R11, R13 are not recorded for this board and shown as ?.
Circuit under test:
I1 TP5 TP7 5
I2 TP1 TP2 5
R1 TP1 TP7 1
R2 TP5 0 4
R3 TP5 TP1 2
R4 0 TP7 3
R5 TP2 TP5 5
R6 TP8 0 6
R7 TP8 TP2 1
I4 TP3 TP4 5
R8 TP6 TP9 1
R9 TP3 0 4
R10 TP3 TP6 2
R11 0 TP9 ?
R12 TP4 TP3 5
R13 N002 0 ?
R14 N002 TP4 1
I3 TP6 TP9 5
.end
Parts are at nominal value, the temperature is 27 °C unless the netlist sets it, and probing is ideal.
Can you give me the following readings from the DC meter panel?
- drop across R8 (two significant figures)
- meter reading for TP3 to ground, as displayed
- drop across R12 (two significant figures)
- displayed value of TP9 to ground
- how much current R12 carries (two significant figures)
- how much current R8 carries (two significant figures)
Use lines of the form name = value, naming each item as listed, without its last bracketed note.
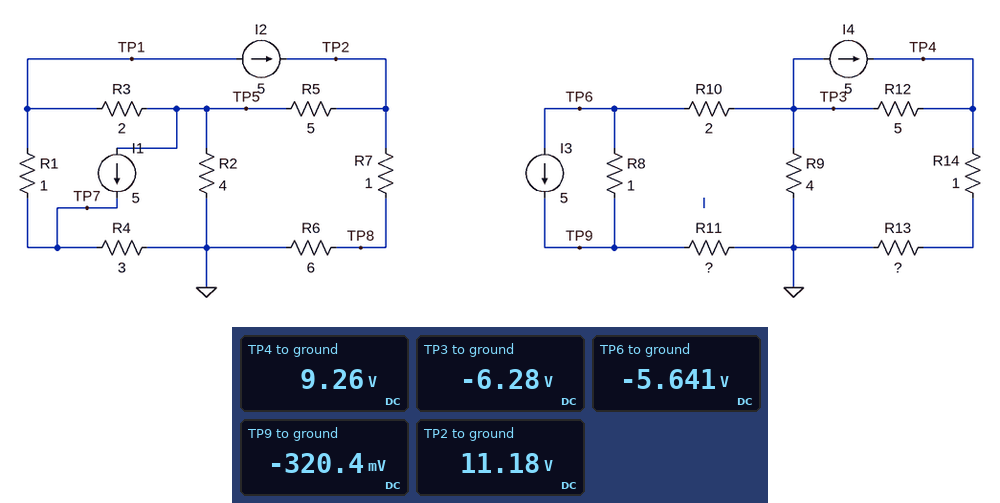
drop across R8 = 5.3 V
meter reading for TP3 to ground, as displayed = -6.28 V
drop across R12 = 16 V
displayed value of TP9 to ground = -320.4 mV
how much current R12 carries = 3.1 A
how much current R8 carries = 5.3 A
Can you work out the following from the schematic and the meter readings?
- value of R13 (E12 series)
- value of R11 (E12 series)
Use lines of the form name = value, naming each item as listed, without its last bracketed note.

value of R13 = 3.9 Ω
value of R11 = 1 Ω
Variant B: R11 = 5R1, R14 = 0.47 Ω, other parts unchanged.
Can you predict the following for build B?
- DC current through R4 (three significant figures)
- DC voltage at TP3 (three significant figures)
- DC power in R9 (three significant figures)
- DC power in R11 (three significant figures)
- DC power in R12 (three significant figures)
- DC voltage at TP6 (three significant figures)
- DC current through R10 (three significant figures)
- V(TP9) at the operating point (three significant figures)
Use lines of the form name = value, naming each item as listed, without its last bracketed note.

DC current through R4 = 139 mA
DC voltage at TP3 = -6.84 V
DC power in R9 = 11.7 W
DC power in R11 = 264 mW
DC power in R12 = 46.9 W
DC voltage at TP6 = -6.39 V
DC current through R10 = 227 mA
V(TP9) at the operating point = -1.16 V
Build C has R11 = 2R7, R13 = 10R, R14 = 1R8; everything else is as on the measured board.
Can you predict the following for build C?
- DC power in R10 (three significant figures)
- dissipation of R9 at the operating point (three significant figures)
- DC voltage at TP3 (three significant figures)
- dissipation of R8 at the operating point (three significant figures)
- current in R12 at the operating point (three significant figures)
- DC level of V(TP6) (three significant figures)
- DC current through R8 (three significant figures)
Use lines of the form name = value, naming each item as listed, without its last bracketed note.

DC power in R10 = 927 µW
dissipation of R9 at the operating point = 5.95 W
DC voltage at TP3 = -4.88 V
dissipation of R8 at the operating point = 24.8 W
current in R12 at the operating point = 3.80 A
DC level of V(TP6) = -4.92 V
DC current through R8 = 4.98 A
